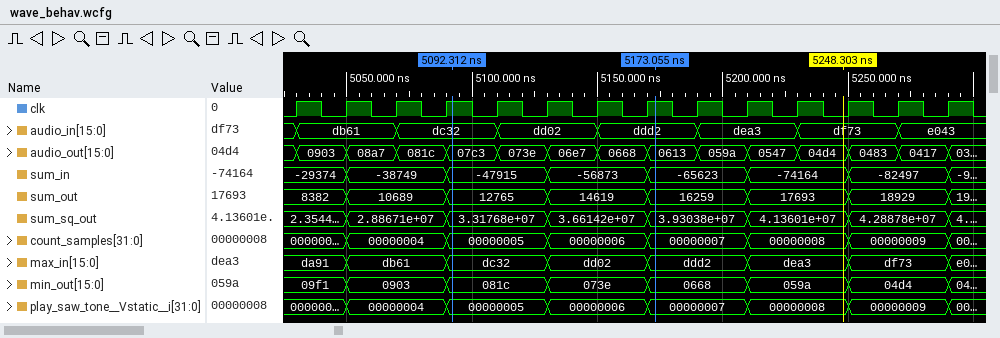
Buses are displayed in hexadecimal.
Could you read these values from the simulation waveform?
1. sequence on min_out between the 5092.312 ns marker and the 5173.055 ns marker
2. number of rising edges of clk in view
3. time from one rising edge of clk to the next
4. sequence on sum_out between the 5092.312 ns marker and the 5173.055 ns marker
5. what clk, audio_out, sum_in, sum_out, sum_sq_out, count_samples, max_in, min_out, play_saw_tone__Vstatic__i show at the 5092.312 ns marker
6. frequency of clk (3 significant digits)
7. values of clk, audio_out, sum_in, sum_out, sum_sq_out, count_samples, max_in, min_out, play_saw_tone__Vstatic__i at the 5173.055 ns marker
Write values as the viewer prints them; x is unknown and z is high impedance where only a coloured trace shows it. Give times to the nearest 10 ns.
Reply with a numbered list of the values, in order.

1. 081c, 073e, 0668
2. 14
3. 20 ns
4. 12765, 14619, 16259
5. clk=1, audio_out=07c3, sum_in=-47915, sum_out=12765, sum_sq_out=3.31768e+07, count_samples=00000005, max_in=dc32, min_out=081c, play_saw_tone__Vstatic__i=00000005
6. 50.0 MHz
7. clk=1, audio_out=0613, sum_in=-65623, sum_out=16259, sum_sq_out=3.93038e+07, count_samples=00000007, max_in=ddd2, min_out=0668, play_saw_tone__Vstatic__i=00000007
